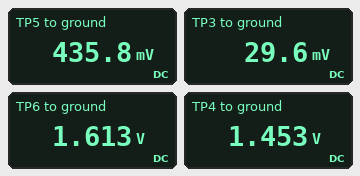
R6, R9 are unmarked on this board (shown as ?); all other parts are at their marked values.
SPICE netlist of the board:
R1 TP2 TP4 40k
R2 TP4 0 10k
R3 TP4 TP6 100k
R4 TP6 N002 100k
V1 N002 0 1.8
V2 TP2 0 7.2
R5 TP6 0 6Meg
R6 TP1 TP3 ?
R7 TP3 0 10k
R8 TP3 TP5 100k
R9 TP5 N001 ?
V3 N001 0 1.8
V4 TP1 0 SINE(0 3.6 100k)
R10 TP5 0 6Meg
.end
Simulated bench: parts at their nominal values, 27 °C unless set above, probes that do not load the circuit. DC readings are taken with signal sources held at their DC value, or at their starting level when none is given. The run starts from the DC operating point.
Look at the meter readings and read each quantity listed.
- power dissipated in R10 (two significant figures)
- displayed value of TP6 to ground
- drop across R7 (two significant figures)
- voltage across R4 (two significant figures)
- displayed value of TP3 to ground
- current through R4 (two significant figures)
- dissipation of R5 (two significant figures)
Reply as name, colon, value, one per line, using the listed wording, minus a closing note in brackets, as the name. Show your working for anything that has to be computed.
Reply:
power dissipated in R10: (435.8 mV)^2 / 6 MΩ = 32 nW
displayed value of TP6 to ground: 1.613 V
drop across R7: 29.6 mV = 30 mV
voltage across R4: 1.8 V - 1.613 V = 190 mV
displayed value of TP3 to ground: 29.6 mV
current through R4: (1.8 V - 1.613 V) / 100 kΩ = 1.9 µA
dissipation of R5: (1.613 V)^2 / 6 MΩ = 430 nW
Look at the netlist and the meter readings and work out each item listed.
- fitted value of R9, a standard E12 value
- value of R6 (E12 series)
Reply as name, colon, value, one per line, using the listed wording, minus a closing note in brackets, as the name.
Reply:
fitted value of R9, a standard E12 value: 330 kΩ
value of R6: 27 kΩ
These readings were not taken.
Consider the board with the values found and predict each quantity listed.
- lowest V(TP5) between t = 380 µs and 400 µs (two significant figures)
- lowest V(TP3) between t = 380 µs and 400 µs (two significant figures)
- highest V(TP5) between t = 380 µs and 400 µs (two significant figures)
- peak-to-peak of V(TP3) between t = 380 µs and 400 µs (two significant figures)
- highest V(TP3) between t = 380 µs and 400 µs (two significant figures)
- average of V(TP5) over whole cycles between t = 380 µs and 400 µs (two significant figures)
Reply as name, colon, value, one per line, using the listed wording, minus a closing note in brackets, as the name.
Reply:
lowest V(TP5) between t = 380 µs and 400 µs: -290 mV
lowest V(TP3) between t = 380 µs and 400 µs: -930 mV
highest V(TP5) between t = 380 µs and 400 µs: 1.2 V
peak-to-peak of V(TP3) between t = 380 µs and 400 µs: 1.9 V
highest V(TP3) between t = 380 µs and 400 µs: 990 mV
average of V(TP5) over whole cycles between t = 380 µs and 400 µs: 440 mV
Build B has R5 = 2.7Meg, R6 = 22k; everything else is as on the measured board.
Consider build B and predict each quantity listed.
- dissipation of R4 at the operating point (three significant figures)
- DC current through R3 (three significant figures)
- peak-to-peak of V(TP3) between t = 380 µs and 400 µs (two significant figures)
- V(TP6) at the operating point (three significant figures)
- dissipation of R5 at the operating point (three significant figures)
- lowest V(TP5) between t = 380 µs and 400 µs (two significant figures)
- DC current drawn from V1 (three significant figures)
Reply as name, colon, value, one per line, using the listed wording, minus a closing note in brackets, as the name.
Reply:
dissipation of R4 at the operating point: 415 nW
DC current through R3: 1.45 µA
peak-to-peak of V(TP3) between t = 380 µs and 400 µs: 2.2 V
V(TP6) at the operating point: 1.60 V
dissipation of R5 at the operating point: 944 nW
lowest V(TP5) between t = 380 µs and 400 µs: -400 mV
DC current drawn from V1: 2.04 µA
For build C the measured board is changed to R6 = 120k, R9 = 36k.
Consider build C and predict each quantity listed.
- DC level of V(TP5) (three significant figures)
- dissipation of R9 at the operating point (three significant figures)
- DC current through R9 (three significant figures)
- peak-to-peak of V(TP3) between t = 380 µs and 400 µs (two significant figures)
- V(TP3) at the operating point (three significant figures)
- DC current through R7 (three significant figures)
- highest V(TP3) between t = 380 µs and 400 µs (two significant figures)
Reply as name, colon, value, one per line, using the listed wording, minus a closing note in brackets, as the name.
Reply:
DC level of V(TP5): 1.35 V
dissipation of R9 at the operating point: 5.68 µW
DC current through R9: 12.6 µA
peak-to-peak of V(TP3) between t = 380 µs and 400 µs: 520 mV
V(TP3) at the operating point: 114 mV
DC current through R7: 11.4 µA
highest V(TP3) between t = 380 µs and 400 µs: 370 mV
